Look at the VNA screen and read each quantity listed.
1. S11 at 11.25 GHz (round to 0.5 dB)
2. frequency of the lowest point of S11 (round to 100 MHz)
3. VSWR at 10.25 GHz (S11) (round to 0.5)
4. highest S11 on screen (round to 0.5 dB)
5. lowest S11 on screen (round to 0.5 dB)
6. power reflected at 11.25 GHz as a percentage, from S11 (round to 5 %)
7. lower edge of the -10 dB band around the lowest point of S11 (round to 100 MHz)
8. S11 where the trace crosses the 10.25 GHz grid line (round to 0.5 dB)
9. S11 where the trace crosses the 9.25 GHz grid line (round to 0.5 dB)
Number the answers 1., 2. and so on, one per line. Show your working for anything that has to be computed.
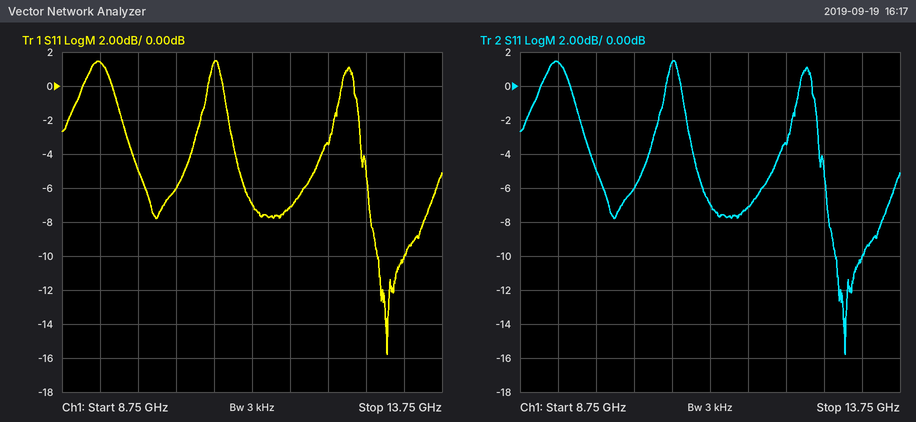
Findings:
1. -7.0 dB
2. 13.0 GHz
3. |Γ| = 10^(-6/20) = 0.5012; VSWR = (1 + 0.5012)/(1 − 0.5012) ≈ 3.0
4. 1.5 dB
5. -16.0 dB
6. 10^(-7/10) ≈ 20 %
7. 12.9 GHz
8. -6.0 dB
9. 1.5 dB
